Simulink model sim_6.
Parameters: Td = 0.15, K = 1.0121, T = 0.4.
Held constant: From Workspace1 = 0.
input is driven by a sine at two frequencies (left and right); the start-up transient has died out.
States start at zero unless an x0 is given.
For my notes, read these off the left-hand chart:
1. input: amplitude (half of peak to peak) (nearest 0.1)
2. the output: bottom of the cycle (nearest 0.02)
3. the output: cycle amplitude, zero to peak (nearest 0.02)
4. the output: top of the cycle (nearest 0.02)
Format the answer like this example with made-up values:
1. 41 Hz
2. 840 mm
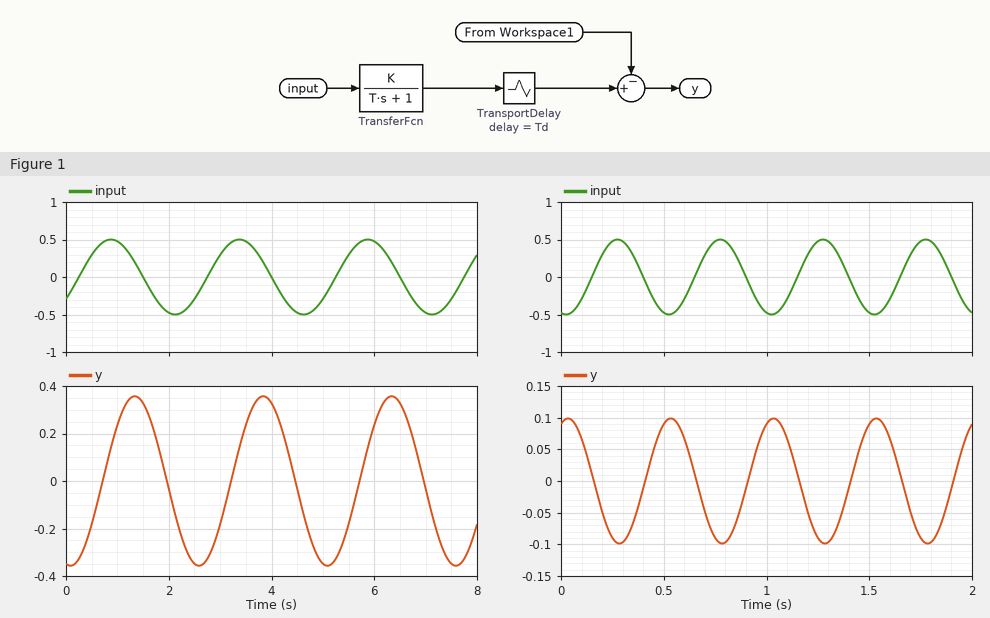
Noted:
1. 0.5
2. -0.36
3. 0.36
4. 0.36
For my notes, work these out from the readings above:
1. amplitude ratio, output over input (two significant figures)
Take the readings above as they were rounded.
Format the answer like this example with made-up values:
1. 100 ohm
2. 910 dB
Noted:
1. 0.72
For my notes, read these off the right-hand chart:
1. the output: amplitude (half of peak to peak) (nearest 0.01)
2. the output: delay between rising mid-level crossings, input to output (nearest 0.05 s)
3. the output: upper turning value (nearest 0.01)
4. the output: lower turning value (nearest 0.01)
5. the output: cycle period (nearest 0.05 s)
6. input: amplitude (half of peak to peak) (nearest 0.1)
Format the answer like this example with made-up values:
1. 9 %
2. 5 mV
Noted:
1. 0.10
2. 0.25 s
3. 0.10
4. -0.10
5. 0.50 s
6. 0.5
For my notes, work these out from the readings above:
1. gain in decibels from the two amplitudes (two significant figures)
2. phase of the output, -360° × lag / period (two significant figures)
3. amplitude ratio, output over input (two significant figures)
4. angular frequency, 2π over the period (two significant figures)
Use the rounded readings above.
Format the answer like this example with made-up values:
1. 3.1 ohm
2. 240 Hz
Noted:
1. -14 dB
2. -180°
3. 0.20
4. 13 rad/s
